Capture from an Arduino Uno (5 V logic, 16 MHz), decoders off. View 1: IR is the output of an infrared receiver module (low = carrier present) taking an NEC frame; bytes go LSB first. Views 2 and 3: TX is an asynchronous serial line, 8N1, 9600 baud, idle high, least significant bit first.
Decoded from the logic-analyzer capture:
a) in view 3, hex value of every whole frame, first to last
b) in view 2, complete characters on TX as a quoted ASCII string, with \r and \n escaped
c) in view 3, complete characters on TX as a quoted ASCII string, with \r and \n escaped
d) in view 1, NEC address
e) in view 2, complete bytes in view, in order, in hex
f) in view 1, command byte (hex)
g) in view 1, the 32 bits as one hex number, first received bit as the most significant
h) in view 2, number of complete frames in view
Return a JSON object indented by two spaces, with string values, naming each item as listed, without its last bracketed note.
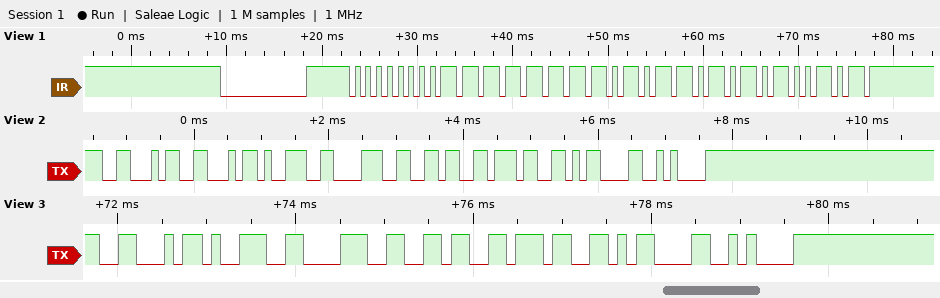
{
  "in view 3, hex value of every whole frame, first to last": "46 39 38 36 37 0D 0A",
  "in view 2, complete characters on TX as a quoted ASCII string, with \\r and \\n escaped": "\"FF9867\\r\\n\"",
  "in view 3, complete characters on TX as a quoted ASCII string, with \\r and \\n escaped": "\"F9867\\r\\n\"",
  "in view 1, NEC address": "0x00",
  "in view 2, complete bytes in view, in order, in hex": "46 46 39 38 36 37 0D 0A",
  "in view 1, command byte": "0x5A",
  "in view 1, the 32 bits as one hex number, first received bit as the most significant": "0x00FF5AA5",
  "in view 2, number of complete frames in view": "8"
}
